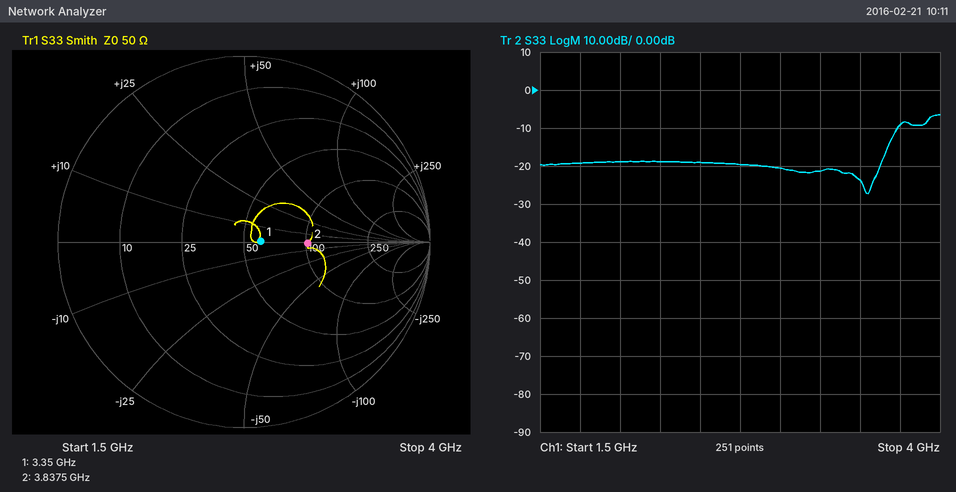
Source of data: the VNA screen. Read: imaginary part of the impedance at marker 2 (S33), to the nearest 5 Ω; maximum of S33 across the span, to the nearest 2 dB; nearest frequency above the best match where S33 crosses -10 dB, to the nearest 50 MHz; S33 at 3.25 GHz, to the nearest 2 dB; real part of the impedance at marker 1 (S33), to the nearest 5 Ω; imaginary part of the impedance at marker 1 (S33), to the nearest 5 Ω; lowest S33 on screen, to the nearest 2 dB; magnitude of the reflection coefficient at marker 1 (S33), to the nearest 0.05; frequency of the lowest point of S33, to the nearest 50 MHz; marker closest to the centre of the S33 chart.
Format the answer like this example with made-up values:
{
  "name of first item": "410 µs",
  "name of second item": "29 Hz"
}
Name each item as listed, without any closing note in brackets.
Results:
{
  "imaginary part of the impedance at marker 2 (S33), to the nearest 5 Ω": "0 Ω",
  "maximum of S33 across the span, to the nearest 2 dB": "-6 dB",
  "nearest frequency above the best match where S33 crosses -10 dB, to the nearest 50 MHz": "3.75 GHz",
  "S33 at 3.25 GHz, to the nearest 2 dB": "-22 dB",
  "real part of the impedance at marker 1 (S33), to the nearest 5 Ω": "60 Ω",
  "imaginary part of the impedance at marker 1 (S33), to the nearest 5 Ω": "0 Ω",
  "lowest S33 on screen, to the nearest 2 dB": "-28 dB",
  "magnitude of the reflection coefficient at marker 1 (S33), to the nearest 0.05": "0.10",
  "frequency of the lowest point of S33, to the nearest 50 MHz": "3.55 GHz",
  "marker closest to the centre of the S33 chart": "marker 1"
}
